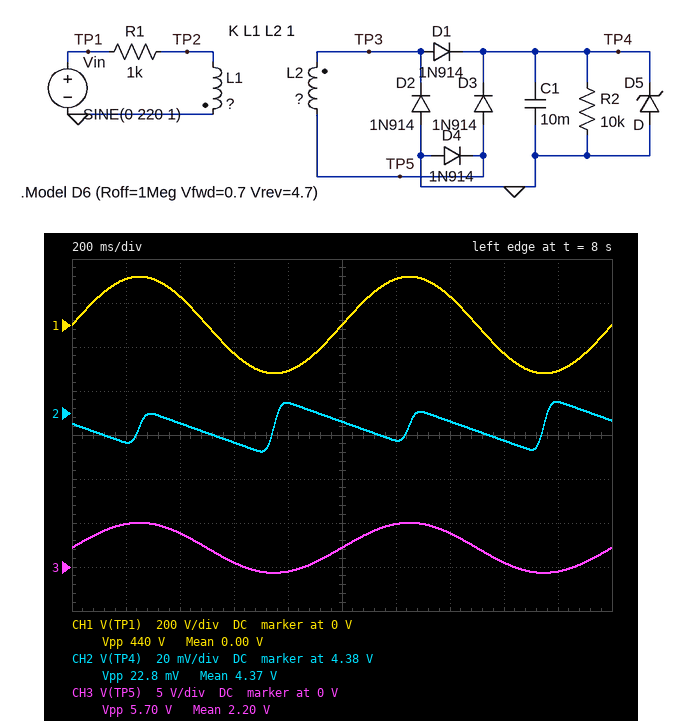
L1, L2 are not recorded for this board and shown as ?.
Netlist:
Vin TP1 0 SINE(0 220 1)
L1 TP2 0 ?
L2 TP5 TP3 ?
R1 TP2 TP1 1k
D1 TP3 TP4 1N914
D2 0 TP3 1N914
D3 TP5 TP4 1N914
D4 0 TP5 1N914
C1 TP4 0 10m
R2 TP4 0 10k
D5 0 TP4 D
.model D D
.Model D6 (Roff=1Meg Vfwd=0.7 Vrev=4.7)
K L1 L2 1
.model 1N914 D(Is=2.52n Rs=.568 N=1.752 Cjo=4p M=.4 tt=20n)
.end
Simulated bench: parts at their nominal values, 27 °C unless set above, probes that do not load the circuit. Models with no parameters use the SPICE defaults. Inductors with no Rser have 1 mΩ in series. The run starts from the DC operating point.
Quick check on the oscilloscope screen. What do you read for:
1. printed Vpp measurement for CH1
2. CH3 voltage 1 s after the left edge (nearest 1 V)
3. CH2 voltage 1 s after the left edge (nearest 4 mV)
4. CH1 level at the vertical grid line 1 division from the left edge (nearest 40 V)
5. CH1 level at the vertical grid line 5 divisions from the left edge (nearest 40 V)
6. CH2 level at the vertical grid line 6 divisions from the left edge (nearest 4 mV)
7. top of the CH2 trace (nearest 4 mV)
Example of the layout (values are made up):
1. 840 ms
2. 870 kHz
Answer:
1. 440 V
2. 2 V
3. 4.376 V
4. 200 V
5. 0 V
6. 4.368 V
7. 4.384 V
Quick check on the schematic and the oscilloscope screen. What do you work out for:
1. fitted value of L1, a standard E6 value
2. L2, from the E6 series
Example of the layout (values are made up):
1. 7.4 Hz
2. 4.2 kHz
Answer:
1. 33 kH
2. 22 H
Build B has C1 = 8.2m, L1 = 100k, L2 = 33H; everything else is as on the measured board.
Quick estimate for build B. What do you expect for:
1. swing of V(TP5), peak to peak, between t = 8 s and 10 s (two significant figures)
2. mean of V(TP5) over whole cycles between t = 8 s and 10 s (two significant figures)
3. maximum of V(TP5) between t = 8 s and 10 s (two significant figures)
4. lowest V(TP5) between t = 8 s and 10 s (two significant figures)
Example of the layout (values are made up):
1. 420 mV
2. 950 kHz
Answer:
1. 4.0 V
2. 1.4 V
3. 3.4 V
4. -630 mV
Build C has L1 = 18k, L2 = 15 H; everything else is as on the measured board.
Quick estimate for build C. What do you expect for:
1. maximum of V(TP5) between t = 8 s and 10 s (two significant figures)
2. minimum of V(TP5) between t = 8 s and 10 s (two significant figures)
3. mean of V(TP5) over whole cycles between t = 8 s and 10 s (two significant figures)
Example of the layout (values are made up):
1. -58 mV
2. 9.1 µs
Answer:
1. 5.7 V
2. -670 mV
3. 2.5 V
